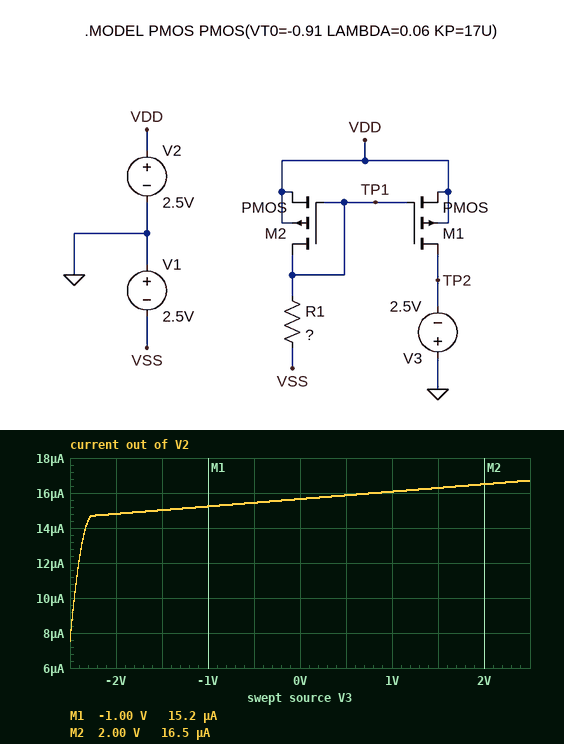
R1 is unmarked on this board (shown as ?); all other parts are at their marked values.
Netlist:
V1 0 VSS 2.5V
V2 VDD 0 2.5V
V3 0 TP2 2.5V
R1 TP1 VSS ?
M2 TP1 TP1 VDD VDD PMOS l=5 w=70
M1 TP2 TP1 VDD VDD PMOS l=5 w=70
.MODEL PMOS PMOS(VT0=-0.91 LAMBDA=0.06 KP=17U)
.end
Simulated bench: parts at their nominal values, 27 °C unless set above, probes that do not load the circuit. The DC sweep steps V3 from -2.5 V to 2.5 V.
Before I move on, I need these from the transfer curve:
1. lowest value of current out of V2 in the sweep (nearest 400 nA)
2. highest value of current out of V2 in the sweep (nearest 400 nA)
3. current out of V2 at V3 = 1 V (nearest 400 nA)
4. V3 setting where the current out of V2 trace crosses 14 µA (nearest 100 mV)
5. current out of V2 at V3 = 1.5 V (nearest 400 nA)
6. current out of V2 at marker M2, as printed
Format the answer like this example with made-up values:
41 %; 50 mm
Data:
7.6 µA; 16.8 µA; 16.0 µA; -2.3 V; 16.4 µA; 16.5 µA
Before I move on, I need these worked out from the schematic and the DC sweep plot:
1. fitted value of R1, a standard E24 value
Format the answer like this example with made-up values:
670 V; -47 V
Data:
510 kΩ
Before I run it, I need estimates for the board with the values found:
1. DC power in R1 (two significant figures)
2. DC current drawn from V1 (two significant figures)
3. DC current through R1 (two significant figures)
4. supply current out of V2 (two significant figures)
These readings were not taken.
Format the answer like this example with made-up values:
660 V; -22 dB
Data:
29 µW; 7.5 µA; 7.5 µA; 17 µA
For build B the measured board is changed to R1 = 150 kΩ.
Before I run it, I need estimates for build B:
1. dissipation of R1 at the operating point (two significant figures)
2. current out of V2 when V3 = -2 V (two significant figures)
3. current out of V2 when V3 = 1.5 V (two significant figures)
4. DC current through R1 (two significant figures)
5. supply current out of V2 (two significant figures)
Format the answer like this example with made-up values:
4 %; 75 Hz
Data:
89 µW; 48 µA; 52 µA; 24 µA; 54 µA
